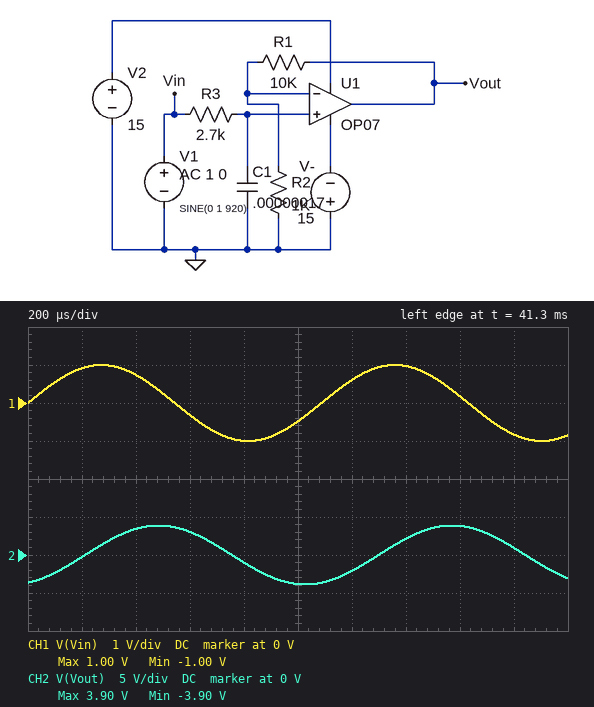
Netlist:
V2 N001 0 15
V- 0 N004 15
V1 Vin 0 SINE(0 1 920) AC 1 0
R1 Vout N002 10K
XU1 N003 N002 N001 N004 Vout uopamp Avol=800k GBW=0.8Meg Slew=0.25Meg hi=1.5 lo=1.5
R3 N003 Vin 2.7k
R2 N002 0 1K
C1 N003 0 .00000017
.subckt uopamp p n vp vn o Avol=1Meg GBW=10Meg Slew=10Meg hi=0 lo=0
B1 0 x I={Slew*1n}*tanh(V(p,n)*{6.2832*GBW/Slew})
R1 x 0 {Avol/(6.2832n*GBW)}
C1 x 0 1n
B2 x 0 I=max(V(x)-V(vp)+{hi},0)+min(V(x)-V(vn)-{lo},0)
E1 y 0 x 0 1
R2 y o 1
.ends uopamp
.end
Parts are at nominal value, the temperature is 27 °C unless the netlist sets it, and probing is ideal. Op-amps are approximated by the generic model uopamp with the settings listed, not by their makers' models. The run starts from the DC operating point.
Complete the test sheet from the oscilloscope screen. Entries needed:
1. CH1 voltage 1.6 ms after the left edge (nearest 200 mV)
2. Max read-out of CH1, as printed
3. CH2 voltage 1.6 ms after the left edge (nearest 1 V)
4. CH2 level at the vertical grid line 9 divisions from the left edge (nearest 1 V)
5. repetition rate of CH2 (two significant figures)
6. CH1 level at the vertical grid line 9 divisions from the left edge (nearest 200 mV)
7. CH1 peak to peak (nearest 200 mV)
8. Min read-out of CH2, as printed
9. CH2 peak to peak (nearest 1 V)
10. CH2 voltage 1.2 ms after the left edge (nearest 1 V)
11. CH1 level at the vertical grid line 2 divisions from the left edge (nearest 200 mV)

200 mV
1.00 V
4 V
1 V
920 Hz
-800 mV
2.0 V
-3.90 V
8 V
-2 V
800 mV
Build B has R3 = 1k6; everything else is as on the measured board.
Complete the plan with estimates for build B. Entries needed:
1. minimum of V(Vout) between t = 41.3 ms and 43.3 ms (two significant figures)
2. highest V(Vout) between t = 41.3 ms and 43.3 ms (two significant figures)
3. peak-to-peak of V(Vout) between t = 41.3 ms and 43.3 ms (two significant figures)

-5.9 V
5.9 V
12 V
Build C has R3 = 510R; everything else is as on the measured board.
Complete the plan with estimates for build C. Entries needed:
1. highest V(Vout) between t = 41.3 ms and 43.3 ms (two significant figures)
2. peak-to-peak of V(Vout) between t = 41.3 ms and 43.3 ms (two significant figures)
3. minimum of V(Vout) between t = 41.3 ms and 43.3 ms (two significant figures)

9.8 V
20 V
-9.8 V
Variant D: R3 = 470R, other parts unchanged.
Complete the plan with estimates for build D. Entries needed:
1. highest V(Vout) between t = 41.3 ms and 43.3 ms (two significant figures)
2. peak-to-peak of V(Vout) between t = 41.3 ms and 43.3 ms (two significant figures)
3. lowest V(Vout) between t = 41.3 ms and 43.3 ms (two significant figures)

10 V
20 V
-10 V
